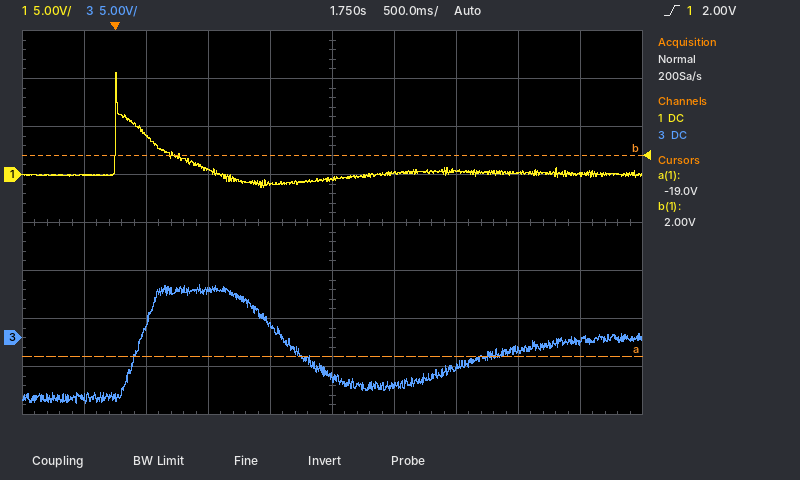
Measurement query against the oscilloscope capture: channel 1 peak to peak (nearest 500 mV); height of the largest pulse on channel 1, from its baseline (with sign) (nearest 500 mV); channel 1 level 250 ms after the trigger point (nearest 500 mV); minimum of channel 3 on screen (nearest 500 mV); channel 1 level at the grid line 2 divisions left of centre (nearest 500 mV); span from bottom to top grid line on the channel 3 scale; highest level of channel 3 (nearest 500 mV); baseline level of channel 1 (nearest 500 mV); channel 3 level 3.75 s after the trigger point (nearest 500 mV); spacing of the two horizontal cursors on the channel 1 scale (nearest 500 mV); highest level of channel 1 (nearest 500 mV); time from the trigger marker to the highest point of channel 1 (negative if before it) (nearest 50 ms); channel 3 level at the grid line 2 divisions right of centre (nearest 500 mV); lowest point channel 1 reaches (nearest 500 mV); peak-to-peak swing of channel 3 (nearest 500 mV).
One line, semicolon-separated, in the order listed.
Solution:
12.0 V; +10.5 V; 4.0 V; -7.0 V; 500 mV; 40 V; 5.5 V; 0.0 V; -500 mV; 21.0 V; 10.5 V; 0 ms; -3.0 V; -1.5 V; 12.5 V
